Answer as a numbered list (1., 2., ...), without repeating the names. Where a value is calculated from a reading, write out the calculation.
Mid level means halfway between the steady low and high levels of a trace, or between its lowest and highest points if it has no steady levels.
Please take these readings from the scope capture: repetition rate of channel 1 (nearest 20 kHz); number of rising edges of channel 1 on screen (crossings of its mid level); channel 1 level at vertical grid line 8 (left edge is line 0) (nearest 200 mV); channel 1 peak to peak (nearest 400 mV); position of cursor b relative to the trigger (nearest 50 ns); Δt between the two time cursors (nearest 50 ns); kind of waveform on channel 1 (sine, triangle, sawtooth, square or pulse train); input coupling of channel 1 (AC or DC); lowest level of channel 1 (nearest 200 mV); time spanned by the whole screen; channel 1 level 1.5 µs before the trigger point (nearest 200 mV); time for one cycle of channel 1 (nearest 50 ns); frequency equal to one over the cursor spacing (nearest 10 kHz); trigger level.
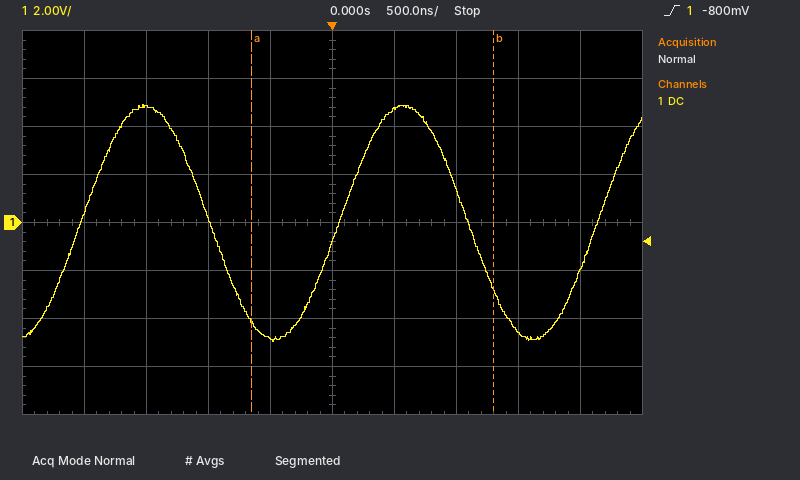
1. 1 / 2.10 µs ≈ 476 kHz, so 480 kHz to the nearest 20 kHz
2. 3
3. -4.6 V
4. 10.0 V
5. +1.30 µs
6. 1.95 µs
7. sine
8. DC
9. -5.0 V
10. 5 µs
11. 4.8 V
12. 2.10 µs
13. 1 / 1.95 µs ≈ 510 kHz
14. -800 mV
